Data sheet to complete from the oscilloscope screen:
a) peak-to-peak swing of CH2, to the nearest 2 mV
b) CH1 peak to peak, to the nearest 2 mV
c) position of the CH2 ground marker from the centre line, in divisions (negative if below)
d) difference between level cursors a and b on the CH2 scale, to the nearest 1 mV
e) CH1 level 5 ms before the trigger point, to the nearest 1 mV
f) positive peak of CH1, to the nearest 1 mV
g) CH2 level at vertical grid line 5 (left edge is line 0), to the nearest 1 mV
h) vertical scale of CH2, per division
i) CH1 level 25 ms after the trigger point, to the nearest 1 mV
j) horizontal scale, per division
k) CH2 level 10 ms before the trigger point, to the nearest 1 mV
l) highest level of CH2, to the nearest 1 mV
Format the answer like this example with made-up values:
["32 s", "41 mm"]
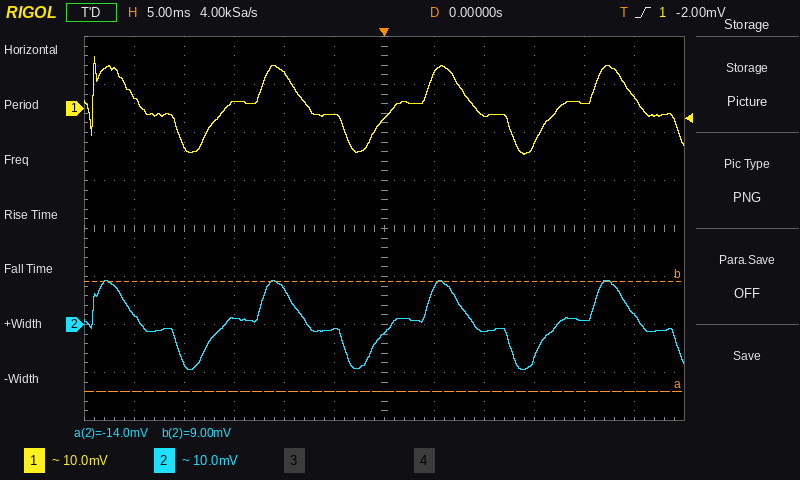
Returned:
["18 mV", "20 mV", "-2.0 div", "23 mV", "-1 mV", "11 mV", "-1 mV", "10 mV", "2 mV", "5 ms", "7 mV", "9 mV"]
